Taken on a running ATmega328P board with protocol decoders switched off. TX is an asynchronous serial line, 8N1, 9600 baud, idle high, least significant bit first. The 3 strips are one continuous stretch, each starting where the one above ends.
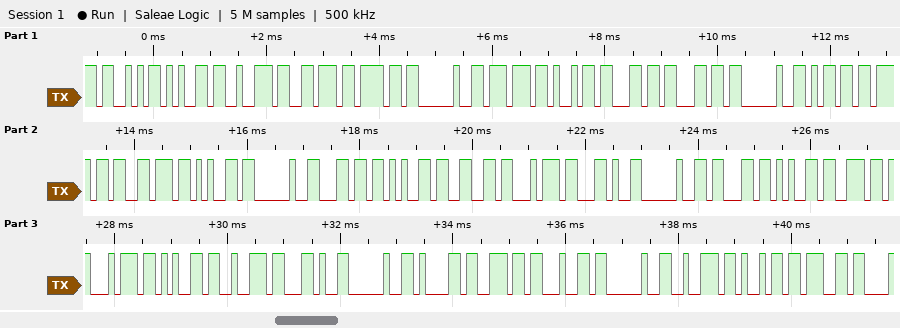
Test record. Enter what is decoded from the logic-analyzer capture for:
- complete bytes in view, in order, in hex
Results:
0x53 0x65 0x72 0x76 0x6F 0x20 0x77 0x69 0x6C 0x6C 0x20 0x6D 0x6F 0x76 0x65 0x20 0x6C 0x65 0x66 0x74 0x2C 0x20 0x63 0x65 0x6E 0x74 0x65 0x72 0x2C 0x20 0x61 0x6E 0x64 0x20 0x72 0x69 0x67
